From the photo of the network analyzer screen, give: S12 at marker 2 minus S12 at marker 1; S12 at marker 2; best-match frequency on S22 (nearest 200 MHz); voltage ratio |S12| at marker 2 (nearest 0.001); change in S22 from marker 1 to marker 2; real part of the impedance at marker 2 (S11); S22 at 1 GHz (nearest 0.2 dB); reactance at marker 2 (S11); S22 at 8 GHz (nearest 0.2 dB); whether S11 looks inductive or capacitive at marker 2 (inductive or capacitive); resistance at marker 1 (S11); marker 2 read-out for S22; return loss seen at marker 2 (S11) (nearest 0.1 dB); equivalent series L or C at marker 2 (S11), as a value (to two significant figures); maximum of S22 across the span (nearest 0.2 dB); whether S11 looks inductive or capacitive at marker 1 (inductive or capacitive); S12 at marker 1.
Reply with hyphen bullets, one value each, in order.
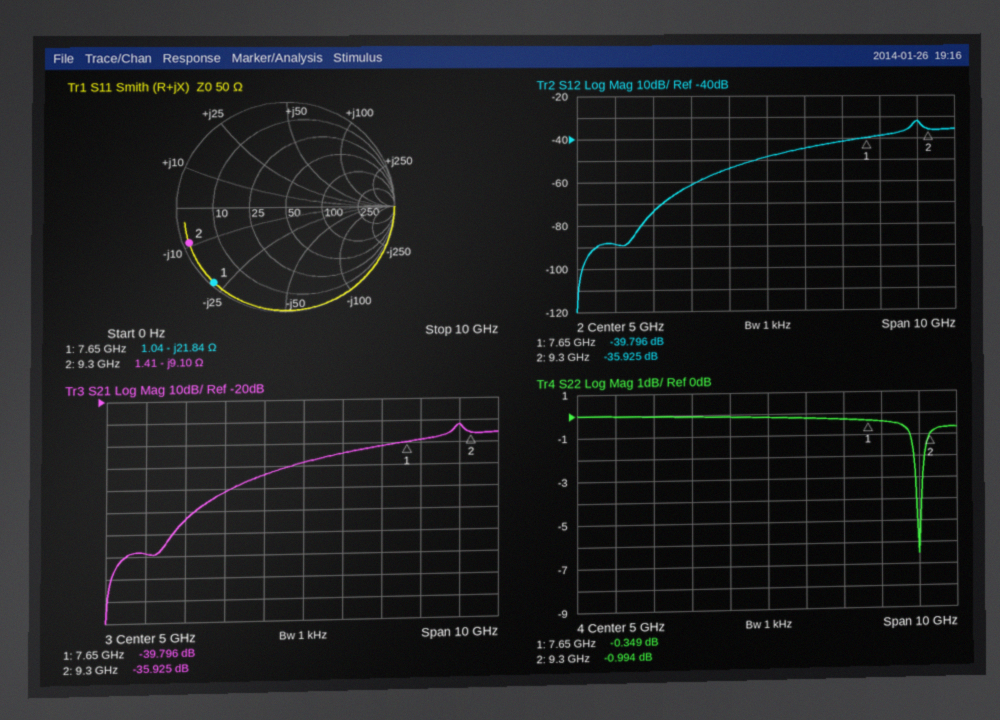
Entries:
- 3.871 dB
- -35.925 dB
- 9.0 GHz
- 0.016
- -0.645 dB
- 1.41 Ω
- 0.0 dB
- -9.10 Ω
- -0.4 dB
- capacitive
- 1.04 Ω
- -0.994 dB
- 0.5 dB
- 1.9 pF
- 0.0 dB
- capacitive
- -39.796 dB
